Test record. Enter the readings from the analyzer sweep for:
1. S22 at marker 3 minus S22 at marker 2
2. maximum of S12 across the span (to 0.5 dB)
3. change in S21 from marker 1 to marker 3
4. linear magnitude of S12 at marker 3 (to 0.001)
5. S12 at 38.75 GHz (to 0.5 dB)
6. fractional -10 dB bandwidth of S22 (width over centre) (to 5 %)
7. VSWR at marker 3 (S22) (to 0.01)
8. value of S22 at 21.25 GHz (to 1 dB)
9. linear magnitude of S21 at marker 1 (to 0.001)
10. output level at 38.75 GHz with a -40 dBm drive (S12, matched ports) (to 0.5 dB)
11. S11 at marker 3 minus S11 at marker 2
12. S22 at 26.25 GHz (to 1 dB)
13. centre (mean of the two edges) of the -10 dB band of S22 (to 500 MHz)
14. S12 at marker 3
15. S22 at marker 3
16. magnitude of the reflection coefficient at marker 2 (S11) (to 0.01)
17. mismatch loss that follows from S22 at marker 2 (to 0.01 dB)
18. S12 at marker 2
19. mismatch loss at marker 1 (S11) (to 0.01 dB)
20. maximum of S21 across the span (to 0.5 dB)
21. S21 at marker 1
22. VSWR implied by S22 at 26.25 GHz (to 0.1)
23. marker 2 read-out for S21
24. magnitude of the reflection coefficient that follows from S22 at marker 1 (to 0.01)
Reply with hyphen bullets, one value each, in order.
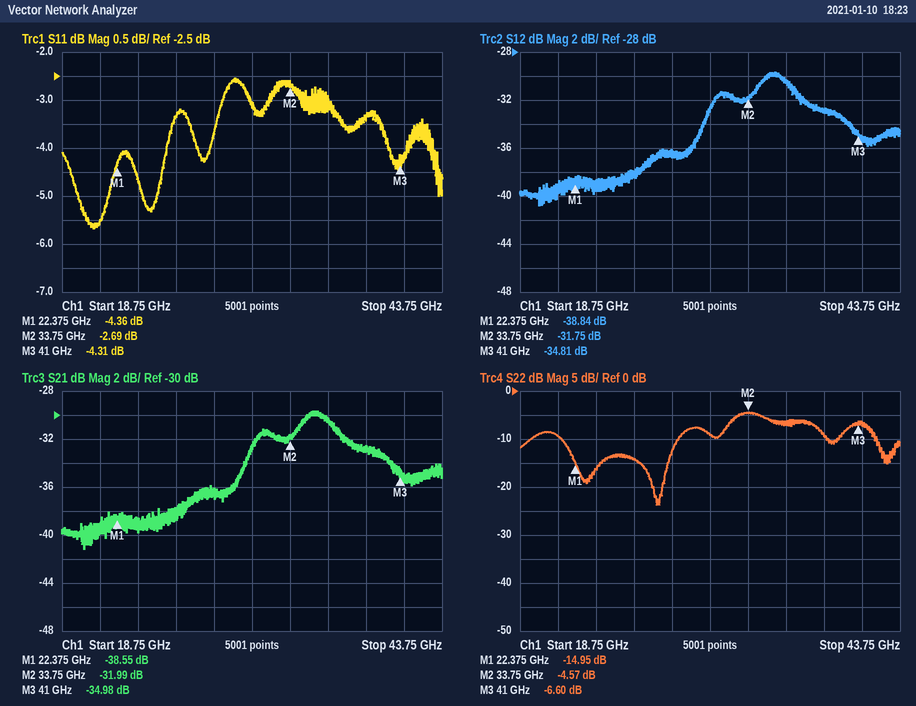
- -2.03 dB
- -29.5 dB
- 3.57 dB
- 0.018
- -33.0 dB
- 30 %
- 2.76
- -9 dB
- 0.012
- -73.0 dBm
- -1.62 dB
- -14 dB
- 25.5 GHz
- -34.81 dB
- -6.60 dB
- 0.73
- 1.87 dB
- -31.75 dB
- 1.98 dB
- -29.5 dB
- -38.55 dB
- 1.5
- -31.99 dB
- 0.18
